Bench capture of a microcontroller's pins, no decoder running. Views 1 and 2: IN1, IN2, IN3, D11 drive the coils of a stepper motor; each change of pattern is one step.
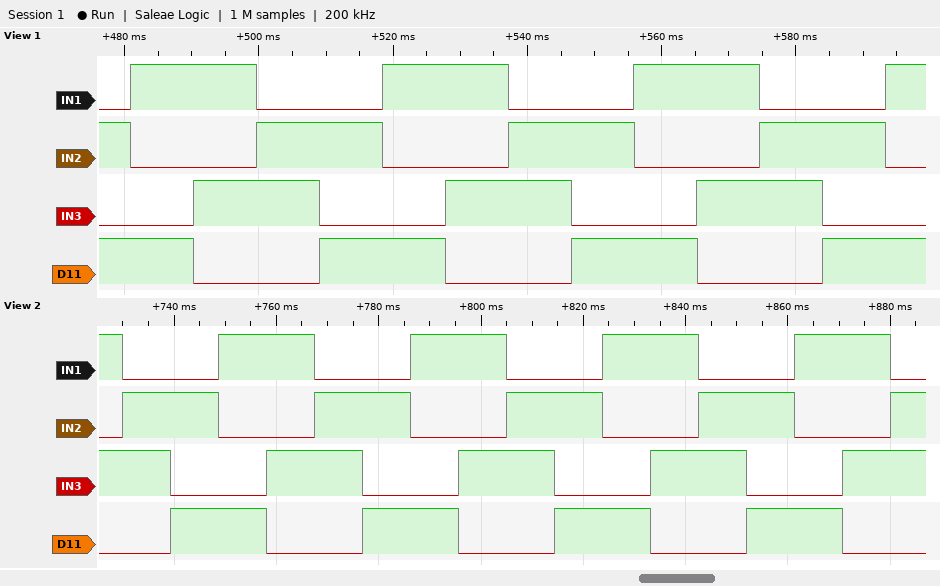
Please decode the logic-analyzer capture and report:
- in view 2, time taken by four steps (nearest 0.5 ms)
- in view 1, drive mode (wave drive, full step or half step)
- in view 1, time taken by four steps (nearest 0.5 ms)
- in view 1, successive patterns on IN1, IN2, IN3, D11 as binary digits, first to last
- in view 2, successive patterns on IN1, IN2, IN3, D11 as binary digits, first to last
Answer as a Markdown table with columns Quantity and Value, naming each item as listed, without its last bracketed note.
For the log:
| Quantity | Value |
|---|---|
| in view 2, time taken by four steps | 37.5 ms |
| in view 1, drive mode | full step |
| in view 1, time taken by four steps | 37.5 ms |
| in view 1, successive patterns on IN1, IN2, IN3, D11 as binary digits, first to last | 0101 1001 1010 0110 0101 1001 1010 0110 0101 1001 1010 0110 0101 1001 |
| in view 2, successive patterns on IN1, IN2, IN3, D11 as binary digits, first to last | 1010 0110 0101 1001 1010 0110 0101 1001 1010 0110 0101 1001 1010 0110 0101 1001 1010 0110 |
